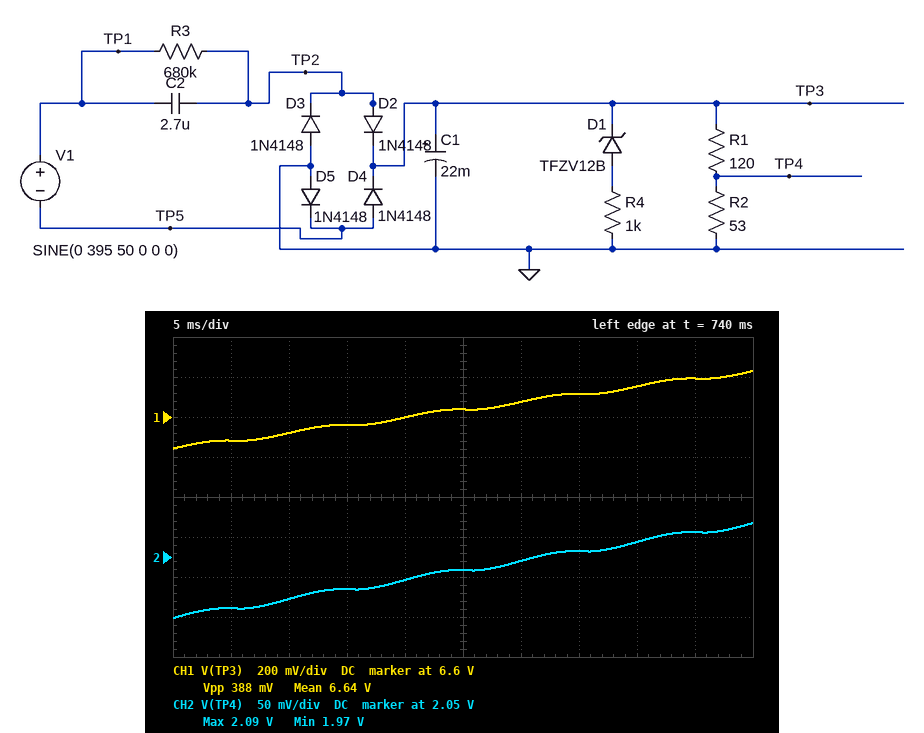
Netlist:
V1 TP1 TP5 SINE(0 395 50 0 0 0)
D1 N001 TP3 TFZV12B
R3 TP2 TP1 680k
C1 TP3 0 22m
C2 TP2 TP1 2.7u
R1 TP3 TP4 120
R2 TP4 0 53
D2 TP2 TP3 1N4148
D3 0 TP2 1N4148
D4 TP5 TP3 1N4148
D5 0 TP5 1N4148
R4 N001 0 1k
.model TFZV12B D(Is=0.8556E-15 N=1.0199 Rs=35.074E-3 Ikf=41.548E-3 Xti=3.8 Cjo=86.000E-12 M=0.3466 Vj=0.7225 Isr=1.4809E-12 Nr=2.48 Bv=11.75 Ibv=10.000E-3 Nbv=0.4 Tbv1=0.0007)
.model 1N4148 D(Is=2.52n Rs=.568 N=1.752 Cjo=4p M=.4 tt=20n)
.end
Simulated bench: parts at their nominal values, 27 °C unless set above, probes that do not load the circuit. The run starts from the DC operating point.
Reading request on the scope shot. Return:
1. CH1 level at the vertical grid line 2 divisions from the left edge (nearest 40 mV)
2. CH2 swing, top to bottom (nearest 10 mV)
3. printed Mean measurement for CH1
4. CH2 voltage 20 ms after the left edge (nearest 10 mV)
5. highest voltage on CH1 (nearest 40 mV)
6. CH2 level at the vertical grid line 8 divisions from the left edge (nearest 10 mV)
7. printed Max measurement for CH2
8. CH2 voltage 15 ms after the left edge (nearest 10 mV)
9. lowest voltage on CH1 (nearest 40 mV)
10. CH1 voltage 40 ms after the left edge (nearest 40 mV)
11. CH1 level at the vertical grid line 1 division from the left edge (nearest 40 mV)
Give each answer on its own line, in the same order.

6.52 V
120 mV
6.64 V
2.02 V
6.84 V
2.07 V
2.09 V
2.01 V
6.44 V
6.76 V
6.48 V
